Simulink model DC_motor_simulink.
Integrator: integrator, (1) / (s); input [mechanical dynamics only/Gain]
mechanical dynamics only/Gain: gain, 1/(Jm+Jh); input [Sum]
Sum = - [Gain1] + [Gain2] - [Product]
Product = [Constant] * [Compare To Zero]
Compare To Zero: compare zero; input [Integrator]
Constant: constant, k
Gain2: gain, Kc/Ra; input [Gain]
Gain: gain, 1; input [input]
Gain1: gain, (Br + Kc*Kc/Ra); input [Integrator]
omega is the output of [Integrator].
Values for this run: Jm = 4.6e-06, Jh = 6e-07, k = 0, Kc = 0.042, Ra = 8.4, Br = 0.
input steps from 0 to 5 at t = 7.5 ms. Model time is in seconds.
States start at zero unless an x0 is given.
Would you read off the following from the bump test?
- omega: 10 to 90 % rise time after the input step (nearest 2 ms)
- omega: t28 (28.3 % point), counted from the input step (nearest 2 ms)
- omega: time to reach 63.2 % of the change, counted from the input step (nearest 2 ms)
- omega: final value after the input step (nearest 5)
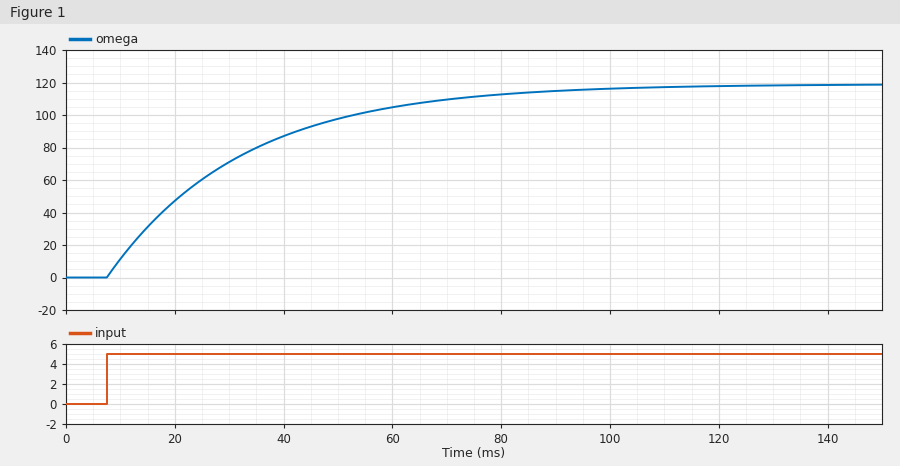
54 ms
8 ms
24 ms
120
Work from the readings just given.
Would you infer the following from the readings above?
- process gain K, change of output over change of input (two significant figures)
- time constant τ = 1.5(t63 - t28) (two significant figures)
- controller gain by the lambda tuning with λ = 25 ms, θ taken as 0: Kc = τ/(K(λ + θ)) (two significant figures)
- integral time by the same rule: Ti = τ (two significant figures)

24
24 ms
0.040
24 ms
